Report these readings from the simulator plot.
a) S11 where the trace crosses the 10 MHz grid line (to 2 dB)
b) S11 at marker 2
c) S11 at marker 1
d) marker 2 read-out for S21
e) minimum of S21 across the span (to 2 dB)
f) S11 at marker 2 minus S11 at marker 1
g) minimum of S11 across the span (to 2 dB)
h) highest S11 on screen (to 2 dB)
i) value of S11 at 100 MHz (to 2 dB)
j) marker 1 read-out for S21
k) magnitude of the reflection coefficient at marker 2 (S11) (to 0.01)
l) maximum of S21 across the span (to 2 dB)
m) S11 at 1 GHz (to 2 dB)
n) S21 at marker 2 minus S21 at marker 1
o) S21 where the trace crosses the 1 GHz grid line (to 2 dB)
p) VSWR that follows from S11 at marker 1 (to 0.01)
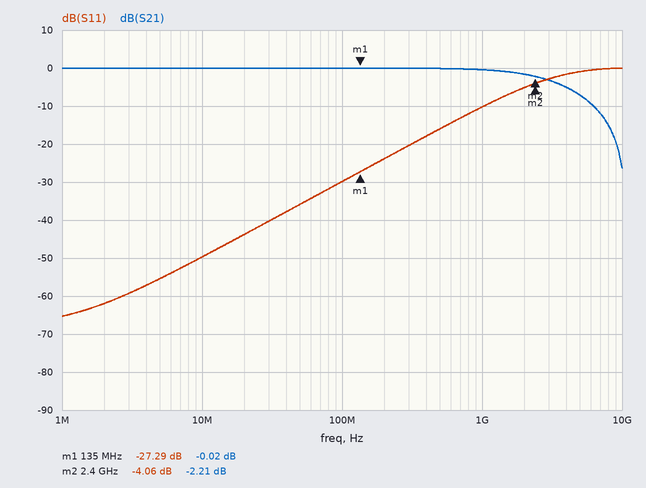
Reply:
-50 dB
-4.06 dB
-27.29 dB
-2.21 dB
-26 dB
23.23 dB
-66 dB
0 dB
-30 dB
-0.02 dB
0.63
0 dB
-10 dB
-2.19 dB
0 dB
1.09
